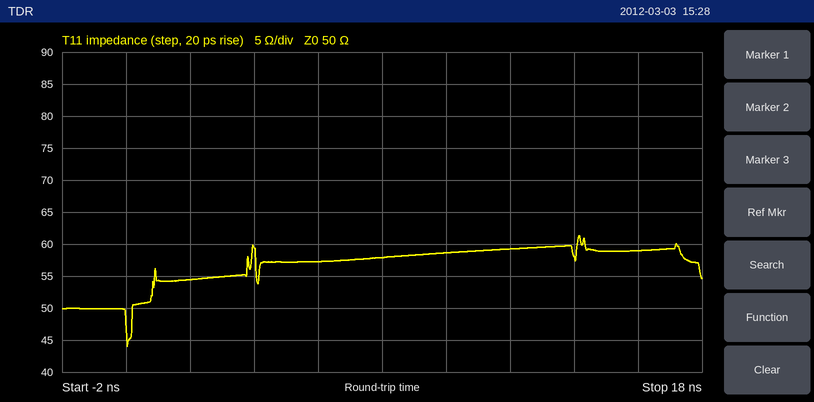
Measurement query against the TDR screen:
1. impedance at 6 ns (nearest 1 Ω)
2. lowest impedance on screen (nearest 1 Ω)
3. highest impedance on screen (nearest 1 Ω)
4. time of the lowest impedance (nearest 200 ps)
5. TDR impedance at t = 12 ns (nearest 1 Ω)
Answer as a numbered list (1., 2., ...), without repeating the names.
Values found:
1. 57 Ω
2. 44 Ω
3. 61 Ω
4. 0.0 ns
5. 59 Ω
